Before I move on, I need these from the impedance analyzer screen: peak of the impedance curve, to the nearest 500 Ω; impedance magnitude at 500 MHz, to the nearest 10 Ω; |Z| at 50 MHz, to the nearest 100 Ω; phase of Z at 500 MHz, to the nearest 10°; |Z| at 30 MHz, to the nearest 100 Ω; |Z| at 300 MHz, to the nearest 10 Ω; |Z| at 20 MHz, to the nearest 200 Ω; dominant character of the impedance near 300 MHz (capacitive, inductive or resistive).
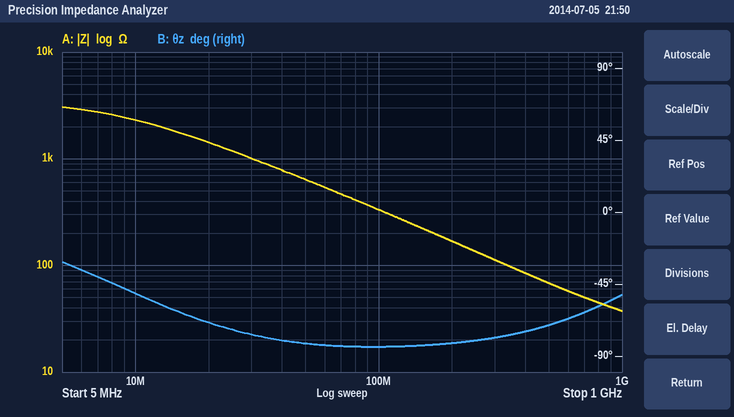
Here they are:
3.0 kΩ
70 Ω
600 Ω
-70°
1.0 kΩ
110 Ω
1.4 kΩ
capacitive
